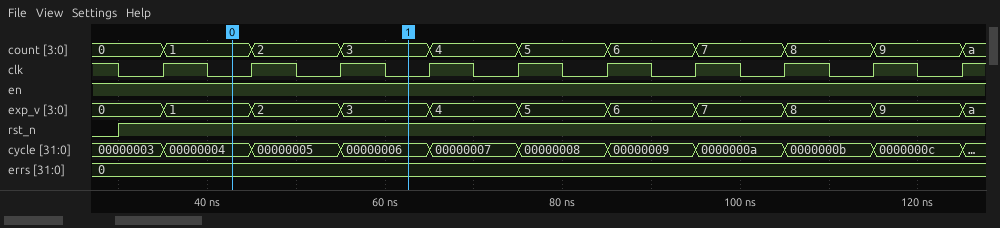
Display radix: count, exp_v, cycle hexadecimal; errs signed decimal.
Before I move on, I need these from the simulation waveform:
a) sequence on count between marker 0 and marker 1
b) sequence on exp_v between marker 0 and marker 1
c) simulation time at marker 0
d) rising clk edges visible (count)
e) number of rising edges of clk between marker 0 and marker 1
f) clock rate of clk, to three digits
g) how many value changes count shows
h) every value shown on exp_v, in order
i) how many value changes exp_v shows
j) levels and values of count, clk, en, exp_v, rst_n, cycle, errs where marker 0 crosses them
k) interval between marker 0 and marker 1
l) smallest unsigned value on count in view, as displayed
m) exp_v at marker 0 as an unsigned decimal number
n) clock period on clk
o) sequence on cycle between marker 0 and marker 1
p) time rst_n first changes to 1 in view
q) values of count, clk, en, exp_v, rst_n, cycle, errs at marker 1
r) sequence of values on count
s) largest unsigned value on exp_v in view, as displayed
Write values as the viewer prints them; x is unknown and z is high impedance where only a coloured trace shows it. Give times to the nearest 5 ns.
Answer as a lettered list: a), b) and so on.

a) 1, 2, 3
b) 1, 2, 3
c) 45 ns
d) 10
e) 2
f) 100 MHz
g) 10
h) 0, 1, 2, 3, 4, 5, 6, 7, 8, 9, a
i) 10
j) count=1, clk=0, en=1, exp_v=1, rst_n=1, cycle=00000004, errs=0
k) 20 ns
l) 0
m) 1
n) 10 ns
o) 00000004, 00000005, 00000006
p) 30 ns
q) count=3, clk=0, en=1, exp_v=3, rst_n=1, cycle=00000006, errs=0
r) 0, 1, 2, 3, 4, 5, 6, 7, 8, 9, a
s) a
